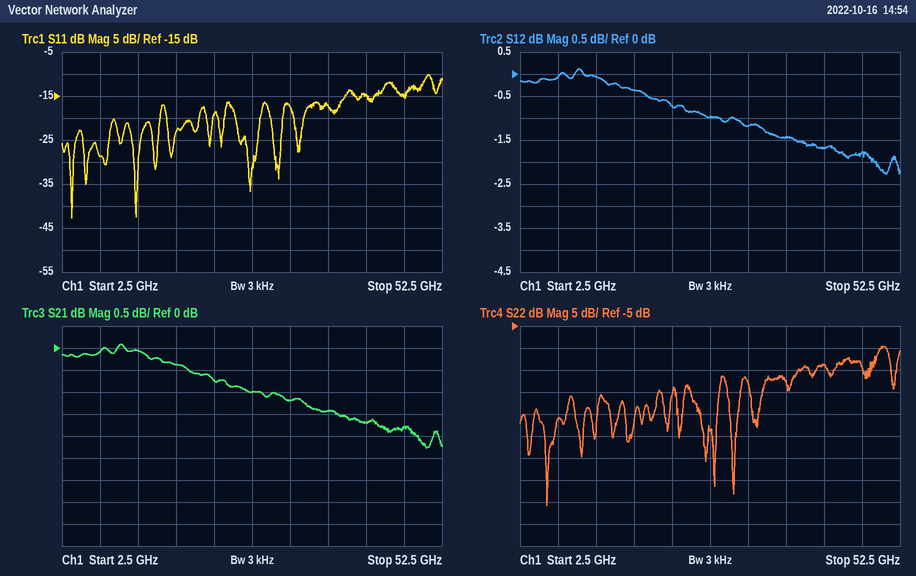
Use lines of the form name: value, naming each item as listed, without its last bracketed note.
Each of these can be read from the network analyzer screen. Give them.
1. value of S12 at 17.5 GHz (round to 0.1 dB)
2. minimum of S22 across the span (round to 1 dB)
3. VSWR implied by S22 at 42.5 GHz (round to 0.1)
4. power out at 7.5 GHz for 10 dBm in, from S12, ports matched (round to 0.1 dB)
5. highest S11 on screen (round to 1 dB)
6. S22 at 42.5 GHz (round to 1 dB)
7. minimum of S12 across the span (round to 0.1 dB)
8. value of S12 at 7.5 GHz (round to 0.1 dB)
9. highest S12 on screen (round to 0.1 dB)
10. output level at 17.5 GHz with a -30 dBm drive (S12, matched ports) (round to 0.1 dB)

value of S12 at 17.5 GHz: -0.4 dB
minimum of S22 across the span: -46 dB
VSWR implied by S22 at 42.5 GHz: 1.5
power out at 7.5 GHz for 10 dBm in, from S12, ports matched: 9.9 dBm
highest S11 on screen: -10 dB
S22 at 42.5 GHz: -14 dB
minimum of S12 across the span: -2.3 dB
value of S12 at 7.5 GHz: -0.1 dB
highest S12 on screen: 0.1 dB
output level at 17.5 GHz with a -30 dBm drive (S12, matched ports): -30.4 dBm
